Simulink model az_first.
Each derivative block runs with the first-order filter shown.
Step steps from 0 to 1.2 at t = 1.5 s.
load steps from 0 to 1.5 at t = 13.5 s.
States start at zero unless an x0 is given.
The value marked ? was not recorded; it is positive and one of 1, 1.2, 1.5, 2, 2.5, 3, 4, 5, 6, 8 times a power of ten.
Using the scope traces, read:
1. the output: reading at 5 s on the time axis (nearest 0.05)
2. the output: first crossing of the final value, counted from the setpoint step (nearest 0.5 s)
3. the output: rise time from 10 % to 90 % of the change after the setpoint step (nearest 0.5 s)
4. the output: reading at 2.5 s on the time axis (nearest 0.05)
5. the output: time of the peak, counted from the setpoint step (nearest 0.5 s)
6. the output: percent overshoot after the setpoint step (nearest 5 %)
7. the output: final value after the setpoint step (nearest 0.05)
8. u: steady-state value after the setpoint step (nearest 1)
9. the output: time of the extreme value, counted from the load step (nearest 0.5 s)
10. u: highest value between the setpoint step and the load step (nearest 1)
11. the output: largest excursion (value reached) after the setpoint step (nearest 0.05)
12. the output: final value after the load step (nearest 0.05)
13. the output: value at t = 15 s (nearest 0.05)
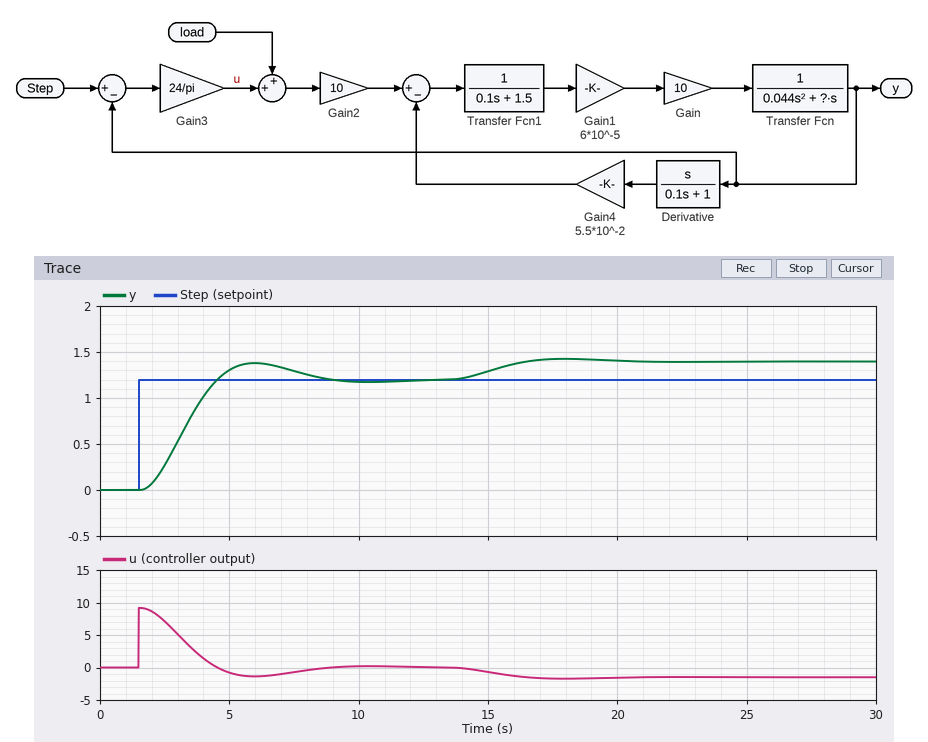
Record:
1.30
3.0 s
2.0 s
0.25
4.5 s
15 %
1.20
0
4.5 s
9
1.40
1.40
1.30
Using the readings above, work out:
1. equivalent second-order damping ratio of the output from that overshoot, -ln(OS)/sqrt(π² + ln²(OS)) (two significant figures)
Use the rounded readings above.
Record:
0.52
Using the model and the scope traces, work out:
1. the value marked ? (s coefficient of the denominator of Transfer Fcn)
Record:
0.04
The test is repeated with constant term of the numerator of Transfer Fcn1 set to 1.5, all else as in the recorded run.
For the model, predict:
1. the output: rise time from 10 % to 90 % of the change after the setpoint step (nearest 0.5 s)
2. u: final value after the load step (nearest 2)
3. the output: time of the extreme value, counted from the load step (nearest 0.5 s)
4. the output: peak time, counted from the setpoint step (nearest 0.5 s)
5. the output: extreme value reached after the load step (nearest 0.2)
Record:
1.5 s
-2
3.5 s
3.5 s
1.4
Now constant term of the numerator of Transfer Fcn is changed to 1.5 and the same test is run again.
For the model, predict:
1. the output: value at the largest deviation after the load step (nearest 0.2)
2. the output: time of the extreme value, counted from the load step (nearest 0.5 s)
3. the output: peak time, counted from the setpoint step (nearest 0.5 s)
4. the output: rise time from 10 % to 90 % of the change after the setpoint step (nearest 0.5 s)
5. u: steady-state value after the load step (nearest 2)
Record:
1.4
3.5 s
3.5 s
1.5 s
-2
